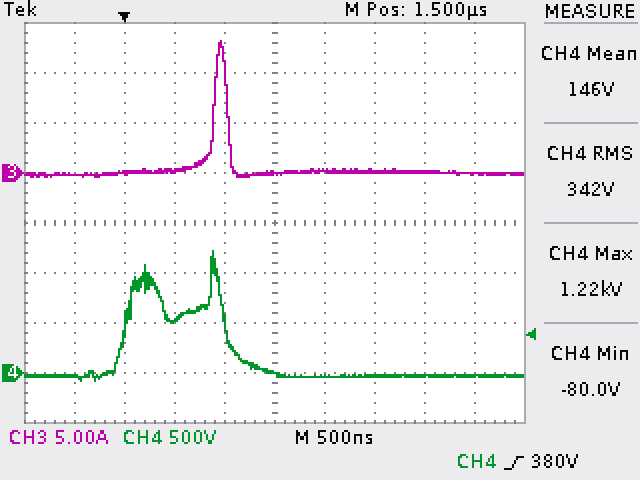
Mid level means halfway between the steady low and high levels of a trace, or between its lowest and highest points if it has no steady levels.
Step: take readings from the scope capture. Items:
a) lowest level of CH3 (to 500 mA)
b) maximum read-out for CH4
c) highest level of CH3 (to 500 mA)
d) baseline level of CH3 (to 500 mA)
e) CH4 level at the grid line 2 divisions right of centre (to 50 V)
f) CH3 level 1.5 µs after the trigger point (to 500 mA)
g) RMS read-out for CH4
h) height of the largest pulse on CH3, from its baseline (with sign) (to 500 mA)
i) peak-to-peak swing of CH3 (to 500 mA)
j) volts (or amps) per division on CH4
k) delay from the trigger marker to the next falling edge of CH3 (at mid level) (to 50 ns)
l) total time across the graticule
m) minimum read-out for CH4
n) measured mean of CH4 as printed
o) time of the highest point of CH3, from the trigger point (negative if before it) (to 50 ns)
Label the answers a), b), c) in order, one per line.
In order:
a) -500 mA
b) 1.22 kV
c) 13.0 A
d) 0.0 A
e) -50 V
f) 0.0 A
g) 342 V
h) +13.0 A
i) 13.5 A
j) 500 V
k) 1.05 µs
l) 5 µs
m) -80.0 V
n) 146 V
o) +950 ns
